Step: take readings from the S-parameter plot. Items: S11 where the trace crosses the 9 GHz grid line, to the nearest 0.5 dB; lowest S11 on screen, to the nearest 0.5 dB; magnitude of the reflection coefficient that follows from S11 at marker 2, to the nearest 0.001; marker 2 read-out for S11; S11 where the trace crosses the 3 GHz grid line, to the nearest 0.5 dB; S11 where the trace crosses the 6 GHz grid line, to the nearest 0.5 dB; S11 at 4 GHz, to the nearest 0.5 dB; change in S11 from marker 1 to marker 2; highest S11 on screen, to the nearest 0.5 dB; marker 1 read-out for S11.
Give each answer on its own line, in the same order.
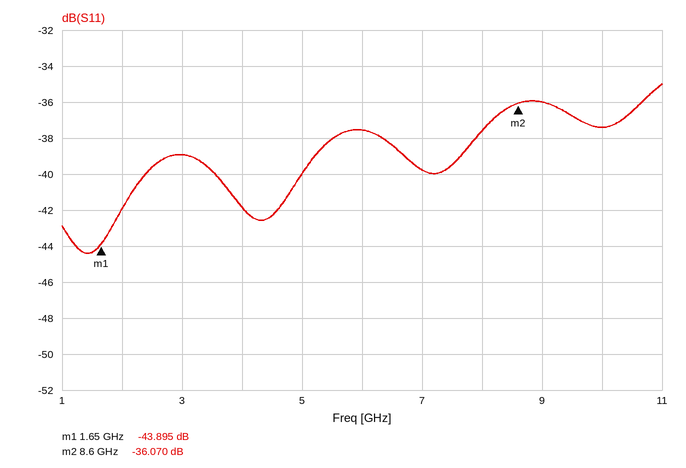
-36.0 dB
-44.5 dB
0.016
-36.070 dB
-39.0 dB
-37.5 dB
-42.0 dB
7.825 dB
-35.0 dB
-43.895 dB
